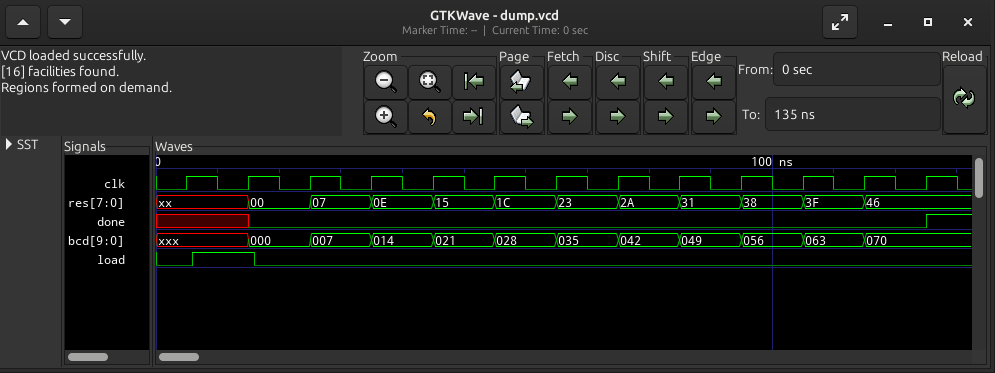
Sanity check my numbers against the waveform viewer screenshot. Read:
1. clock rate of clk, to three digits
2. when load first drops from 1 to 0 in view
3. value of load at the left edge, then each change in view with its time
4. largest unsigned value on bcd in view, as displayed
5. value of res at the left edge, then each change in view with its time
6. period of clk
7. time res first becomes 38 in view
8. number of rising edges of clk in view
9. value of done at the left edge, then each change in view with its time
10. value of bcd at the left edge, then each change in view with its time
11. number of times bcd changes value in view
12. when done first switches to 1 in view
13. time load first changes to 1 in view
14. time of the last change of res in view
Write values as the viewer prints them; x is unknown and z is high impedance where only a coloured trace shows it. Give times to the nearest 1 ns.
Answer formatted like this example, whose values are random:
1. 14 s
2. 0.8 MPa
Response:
1. 100 MHz
2. 16 ns
3. 0, 1 at 6 ns, 0 at 16 ns
4. 070
5. xx, 00 at 15 ns, 07 at 25 ns, 0E at 35 ns, 15 at 45 ns, 1C at 55 ns, 23 at 65 ns, 2A at 75 ns, 31 at 85 ns, 38 at 95 ns, 3F at 105 ns, 46 at 115 ns
6. 10 ns
7. 95 ns
8. 13
9. x, 0 at 15 ns, 1 at 125 ns
10. xxx, 000 at 15 ns, 007 at 25 ns, 014 at 35 ns, 021 at 45 ns, 028 at 55 ns, 035 at 65 ns, 042 at 75 ns, 049 at 85 ns, 056 at 95 ns, 063 at 105 ns, 070 at 115 ns
11. 11
12. 125 ns
13. 6 ns
14. 115 ns
